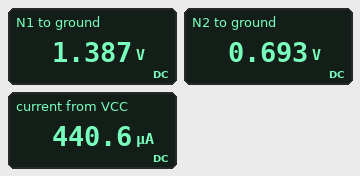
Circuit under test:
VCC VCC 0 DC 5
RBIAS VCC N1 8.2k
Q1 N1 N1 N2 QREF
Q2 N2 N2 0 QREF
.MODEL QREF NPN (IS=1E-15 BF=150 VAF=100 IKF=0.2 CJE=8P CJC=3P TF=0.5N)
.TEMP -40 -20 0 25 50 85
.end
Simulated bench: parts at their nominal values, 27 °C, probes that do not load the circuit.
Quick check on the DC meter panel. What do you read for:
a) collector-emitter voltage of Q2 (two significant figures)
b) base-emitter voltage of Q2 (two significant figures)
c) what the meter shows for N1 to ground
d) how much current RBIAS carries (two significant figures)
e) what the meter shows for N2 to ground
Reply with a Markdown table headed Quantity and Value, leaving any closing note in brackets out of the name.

| Quantity | Value |
|---|---|
| collector-emitter voltage of Q2 | 690 mV |
| base-emitter voltage of Q2 | 690 mV |
| what the meter shows for N1 to ground | 1.387 V |
| how much current RBIAS carries | 440 µA |
| what the meter shows for N2 to ground | 0.693 V |
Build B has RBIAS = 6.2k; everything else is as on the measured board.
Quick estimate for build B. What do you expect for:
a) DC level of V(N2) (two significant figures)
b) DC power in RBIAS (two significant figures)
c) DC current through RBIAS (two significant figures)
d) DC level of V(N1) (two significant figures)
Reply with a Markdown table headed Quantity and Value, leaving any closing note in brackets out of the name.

| Quantity | Value |
|---|---|
| DC level of V(N2) | 700 mV |
| DC power in RBIAS | 2.1 mW |
| DC current through RBIAS | 580 µA |
| DC level of V(N1) | 1.4 V |
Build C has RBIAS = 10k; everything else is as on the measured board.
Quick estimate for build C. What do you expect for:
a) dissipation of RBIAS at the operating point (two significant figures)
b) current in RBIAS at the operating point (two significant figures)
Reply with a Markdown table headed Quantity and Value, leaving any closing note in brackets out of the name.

| Quantity | Value |
|---|---|
| dissipation of RBIAS at the operating point | 1.3 mW |
| current in RBIAS at the operating point | 360 µA |
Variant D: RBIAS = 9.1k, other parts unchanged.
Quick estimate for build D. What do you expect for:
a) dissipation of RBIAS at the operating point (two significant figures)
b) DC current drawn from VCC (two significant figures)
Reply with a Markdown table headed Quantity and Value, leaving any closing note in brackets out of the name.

| Quantity | Value |
|---|---|
| dissipation of RBIAS at the operating point | 1.4 mW |
| DC current drawn from VCC | 400 µA |
